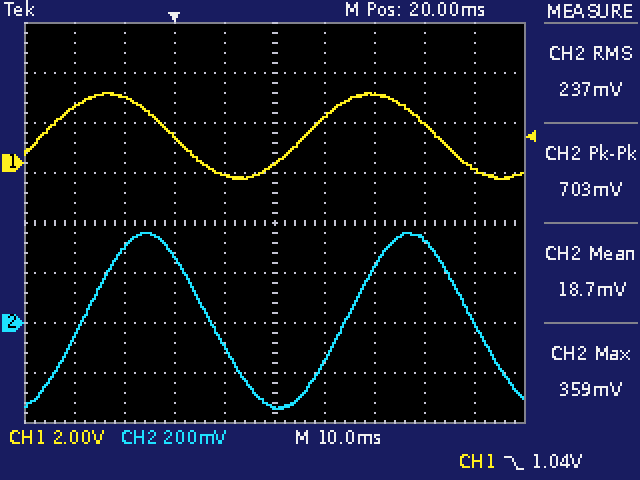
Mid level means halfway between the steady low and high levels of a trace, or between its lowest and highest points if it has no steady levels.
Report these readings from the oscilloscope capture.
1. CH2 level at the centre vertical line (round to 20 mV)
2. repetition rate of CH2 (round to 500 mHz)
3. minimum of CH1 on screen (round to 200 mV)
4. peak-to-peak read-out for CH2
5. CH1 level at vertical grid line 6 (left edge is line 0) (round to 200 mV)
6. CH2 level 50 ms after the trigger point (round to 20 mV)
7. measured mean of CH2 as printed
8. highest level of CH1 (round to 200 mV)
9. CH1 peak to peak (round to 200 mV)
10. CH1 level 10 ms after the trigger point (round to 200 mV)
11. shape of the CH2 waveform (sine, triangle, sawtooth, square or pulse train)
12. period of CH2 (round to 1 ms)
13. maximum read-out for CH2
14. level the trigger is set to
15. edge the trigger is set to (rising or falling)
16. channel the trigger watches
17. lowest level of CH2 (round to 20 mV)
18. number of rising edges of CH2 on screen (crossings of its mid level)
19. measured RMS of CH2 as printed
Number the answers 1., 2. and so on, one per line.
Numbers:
1. -340 mV
2. 19.0 Hz
3. -600 mV
4. 703 mV
5. 1.8 V
6. 340 mV
7. 18.7 mV
8. 2.8 V
9. 3.4 V
10. -400 mV
11. sine
12. 53 ms
13. 359 mV
14. 1.04 V
15. falling
16. CH1
17. -340 mV
18. 2
19. 237 mV
